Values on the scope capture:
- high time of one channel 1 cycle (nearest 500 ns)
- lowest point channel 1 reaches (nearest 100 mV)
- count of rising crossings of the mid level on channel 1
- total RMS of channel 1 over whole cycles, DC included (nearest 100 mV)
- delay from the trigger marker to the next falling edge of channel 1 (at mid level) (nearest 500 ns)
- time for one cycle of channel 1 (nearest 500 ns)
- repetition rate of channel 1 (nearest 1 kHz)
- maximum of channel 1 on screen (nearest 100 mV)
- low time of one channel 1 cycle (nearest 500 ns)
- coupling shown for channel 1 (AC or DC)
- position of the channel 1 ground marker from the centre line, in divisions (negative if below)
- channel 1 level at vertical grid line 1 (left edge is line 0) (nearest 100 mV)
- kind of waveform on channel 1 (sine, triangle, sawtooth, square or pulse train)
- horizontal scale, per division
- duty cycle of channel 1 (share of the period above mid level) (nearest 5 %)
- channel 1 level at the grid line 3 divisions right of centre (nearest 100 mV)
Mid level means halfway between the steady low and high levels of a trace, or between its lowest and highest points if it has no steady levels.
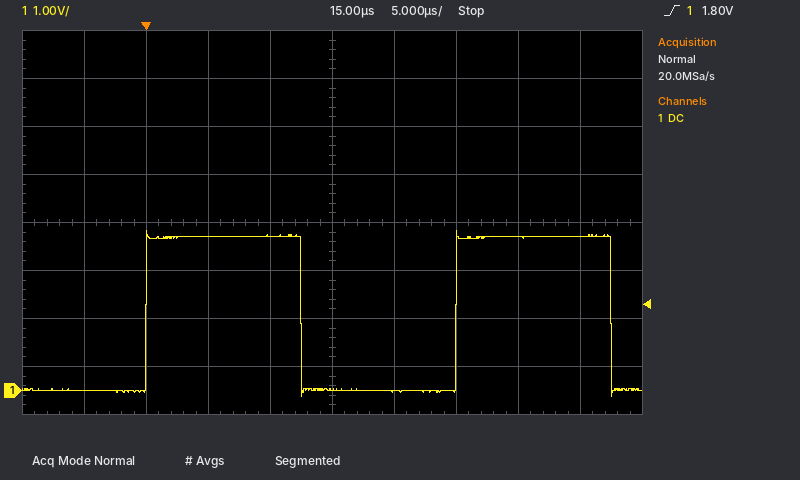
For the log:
12.5 µs
-100 mV
2
2.3 V
12.5 µs
25.0 µs
40 kHz
3.3 V
12.5 µs
DC
-3.5 div
0.0 V
square
5 µs
50 %
3.2 V
